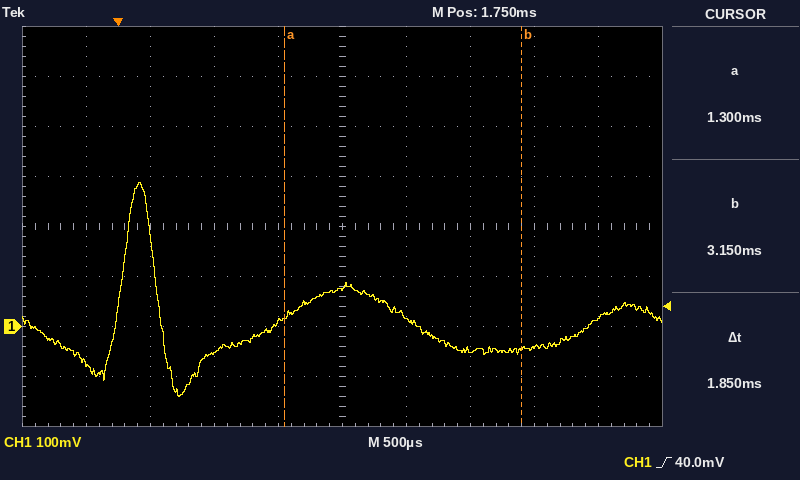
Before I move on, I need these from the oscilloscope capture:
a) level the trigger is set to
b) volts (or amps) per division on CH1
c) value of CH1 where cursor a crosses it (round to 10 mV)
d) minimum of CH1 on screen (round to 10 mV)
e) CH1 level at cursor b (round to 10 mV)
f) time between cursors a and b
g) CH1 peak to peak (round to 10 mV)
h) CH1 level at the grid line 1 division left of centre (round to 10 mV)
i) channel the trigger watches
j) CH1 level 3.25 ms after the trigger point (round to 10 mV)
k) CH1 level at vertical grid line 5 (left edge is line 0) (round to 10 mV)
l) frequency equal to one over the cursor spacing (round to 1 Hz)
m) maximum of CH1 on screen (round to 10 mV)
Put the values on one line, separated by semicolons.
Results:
40.0 mV; 100 mV; 20 mV; -140 mV; -50 mV; 1.85 ms; 430 mV; 10 mV; CH1; -40 mV; 80 mV; 541 Hz; 290 mV
